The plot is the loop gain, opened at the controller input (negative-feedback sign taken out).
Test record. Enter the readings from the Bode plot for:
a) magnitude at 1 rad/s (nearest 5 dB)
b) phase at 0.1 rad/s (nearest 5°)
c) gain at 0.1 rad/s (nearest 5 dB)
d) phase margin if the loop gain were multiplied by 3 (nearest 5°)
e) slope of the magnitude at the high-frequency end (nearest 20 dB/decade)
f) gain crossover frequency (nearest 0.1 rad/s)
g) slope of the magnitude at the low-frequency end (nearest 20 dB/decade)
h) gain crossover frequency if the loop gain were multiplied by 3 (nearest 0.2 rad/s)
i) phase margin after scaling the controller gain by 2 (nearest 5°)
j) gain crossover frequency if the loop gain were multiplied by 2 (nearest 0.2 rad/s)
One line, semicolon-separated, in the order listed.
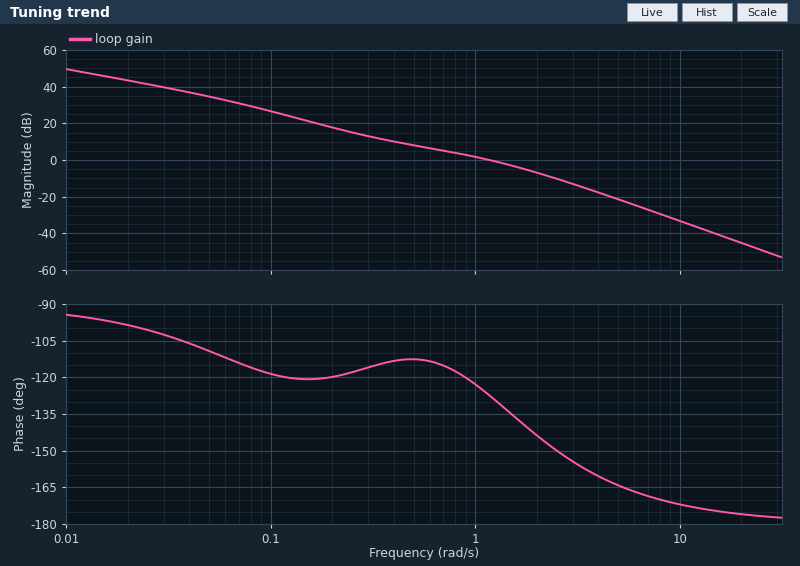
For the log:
0 dB; -120°; 25 dB; 30°; -40 dB/decade; 1.2 rad/s; -20 dB/decade; 2.4 rad/s; 40°; 1.8 rad/s
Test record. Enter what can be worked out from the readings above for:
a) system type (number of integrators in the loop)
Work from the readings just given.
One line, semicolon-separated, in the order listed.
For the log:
1
